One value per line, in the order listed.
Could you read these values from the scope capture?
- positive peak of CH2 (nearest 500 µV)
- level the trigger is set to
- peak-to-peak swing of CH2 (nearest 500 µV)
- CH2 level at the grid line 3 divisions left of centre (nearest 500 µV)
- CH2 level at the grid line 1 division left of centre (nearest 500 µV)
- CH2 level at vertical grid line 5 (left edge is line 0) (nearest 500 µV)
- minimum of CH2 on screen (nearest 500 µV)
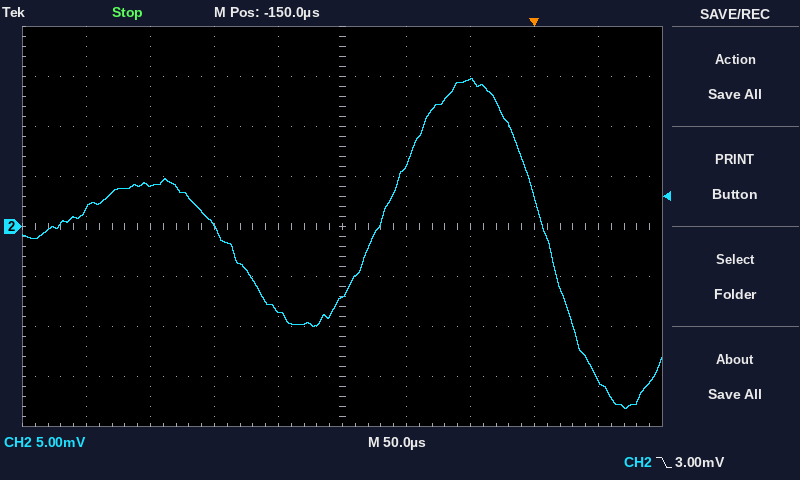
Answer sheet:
15.0 mV
3.00 mV
33.0 mV
4.0 mV
-8.5 mV
-7.0 mV
-18.0 mV
